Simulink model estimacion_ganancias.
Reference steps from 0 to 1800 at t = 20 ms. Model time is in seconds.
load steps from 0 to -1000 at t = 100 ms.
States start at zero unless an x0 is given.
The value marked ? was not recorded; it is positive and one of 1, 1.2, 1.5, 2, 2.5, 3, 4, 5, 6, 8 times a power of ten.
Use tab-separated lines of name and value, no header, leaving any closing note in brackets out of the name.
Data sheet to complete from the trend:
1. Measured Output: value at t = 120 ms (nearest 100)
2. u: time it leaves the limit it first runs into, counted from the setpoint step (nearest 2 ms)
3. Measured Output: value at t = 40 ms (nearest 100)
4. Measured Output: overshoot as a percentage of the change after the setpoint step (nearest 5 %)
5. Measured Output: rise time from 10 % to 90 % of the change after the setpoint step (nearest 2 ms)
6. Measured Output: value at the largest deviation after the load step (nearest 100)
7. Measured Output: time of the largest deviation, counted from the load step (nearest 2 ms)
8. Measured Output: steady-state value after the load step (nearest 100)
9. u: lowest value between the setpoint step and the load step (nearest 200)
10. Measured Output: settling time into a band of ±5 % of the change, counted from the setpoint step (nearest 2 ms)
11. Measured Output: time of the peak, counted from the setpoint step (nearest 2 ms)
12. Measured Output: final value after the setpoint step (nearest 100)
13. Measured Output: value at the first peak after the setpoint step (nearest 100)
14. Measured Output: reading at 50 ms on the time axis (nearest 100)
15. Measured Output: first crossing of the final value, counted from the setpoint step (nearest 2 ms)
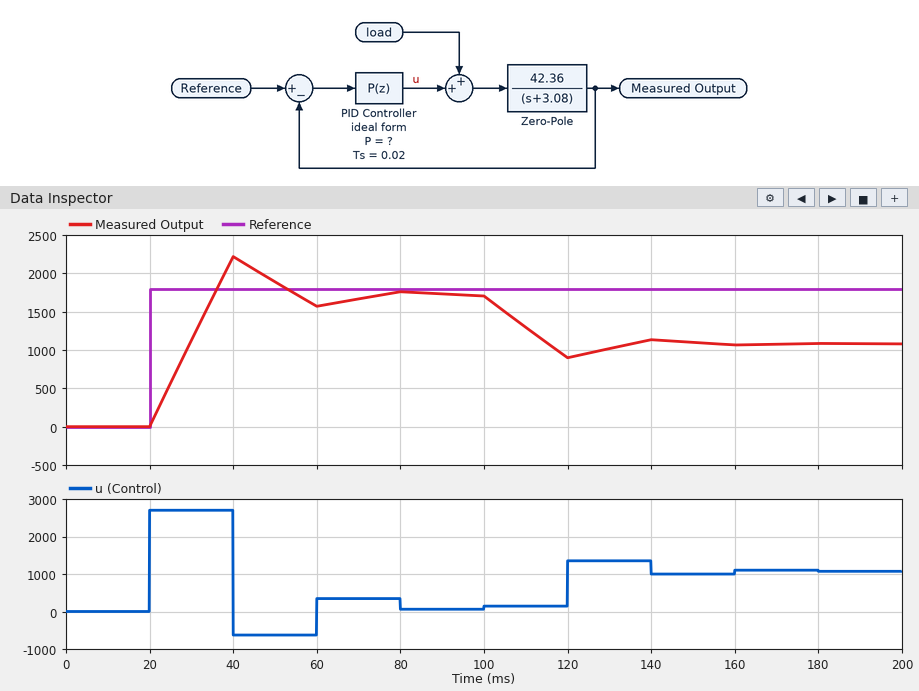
Measured Output: value at t = 120 ms	900
u: time it leaves the limit it first runs into, counted from the setpoint step	20 ms
Measured Output: value at t = 40 ms	2200
Measured Output: overshoot as a percentage of the change after the setpoint step	30 %
Measured Output: rise time from 10 % to 90 % of the change after the setpoint step	12 ms
Measured Output: value at the largest deviation after the load step	900
Measured Output: time of the largest deviation, counted from the load step	20 ms
Measured Output: steady-state value after the load step	1100
u: lowest value between the setpoint step and the load step	-600
Measured Output: settling time into a band of ±5 % of the change, counted from the setpoint step	46 ms
Measured Output: time of the peak, counted from the setpoint step	20 ms
Measured Output: final value after the setpoint step	1700
Measured Output: value at the first peak after the setpoint step	2200
Measured Output: reading at 50 ms on the time axis	1900
Measured Output: first crossing of the final value, counted from the setpoint step	16 ms
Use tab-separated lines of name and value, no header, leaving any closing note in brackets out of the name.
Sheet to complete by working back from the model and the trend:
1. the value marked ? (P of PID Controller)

the value marked ?	1.5
